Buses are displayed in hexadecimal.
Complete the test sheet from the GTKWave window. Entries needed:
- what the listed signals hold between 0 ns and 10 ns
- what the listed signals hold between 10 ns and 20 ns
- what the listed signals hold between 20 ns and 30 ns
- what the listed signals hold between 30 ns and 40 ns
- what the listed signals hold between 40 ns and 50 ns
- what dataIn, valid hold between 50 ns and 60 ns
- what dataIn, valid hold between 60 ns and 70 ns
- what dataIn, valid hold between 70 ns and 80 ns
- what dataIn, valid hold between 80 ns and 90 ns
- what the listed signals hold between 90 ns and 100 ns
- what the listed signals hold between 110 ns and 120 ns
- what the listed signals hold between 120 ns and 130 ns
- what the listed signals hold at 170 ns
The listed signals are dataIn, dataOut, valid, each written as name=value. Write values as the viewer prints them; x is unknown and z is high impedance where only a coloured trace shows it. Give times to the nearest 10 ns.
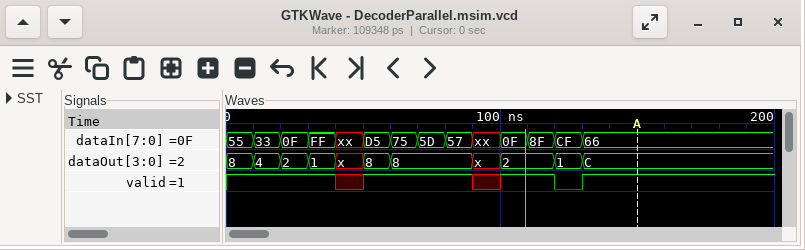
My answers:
dataIn=55, dataOut=8, valid=1
dataIn=33, dataOut=4, valid=1
dataIn=0F, dataOut=2, valid=1
dataIn=FF, dataOut=1, valid=1
dataIn=xx, dataOut=x, valid=x
dataIn=D5, valid=1
dataIn=75, valid=1
dataIn=5D, valid=1
dataIn=57, valid=1
dataIn=xx, dataOut=x, valid=x
dataIn=8F, dataOut=2, valid=1
dataIn=CF, dataOut=1, valid=0
dataIn=66, dataOut=C, valid=1
